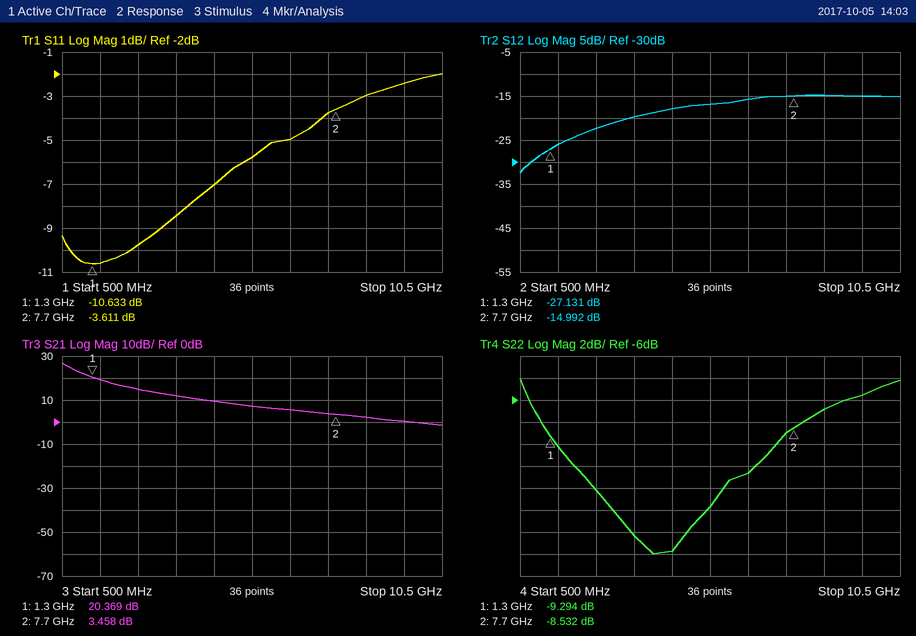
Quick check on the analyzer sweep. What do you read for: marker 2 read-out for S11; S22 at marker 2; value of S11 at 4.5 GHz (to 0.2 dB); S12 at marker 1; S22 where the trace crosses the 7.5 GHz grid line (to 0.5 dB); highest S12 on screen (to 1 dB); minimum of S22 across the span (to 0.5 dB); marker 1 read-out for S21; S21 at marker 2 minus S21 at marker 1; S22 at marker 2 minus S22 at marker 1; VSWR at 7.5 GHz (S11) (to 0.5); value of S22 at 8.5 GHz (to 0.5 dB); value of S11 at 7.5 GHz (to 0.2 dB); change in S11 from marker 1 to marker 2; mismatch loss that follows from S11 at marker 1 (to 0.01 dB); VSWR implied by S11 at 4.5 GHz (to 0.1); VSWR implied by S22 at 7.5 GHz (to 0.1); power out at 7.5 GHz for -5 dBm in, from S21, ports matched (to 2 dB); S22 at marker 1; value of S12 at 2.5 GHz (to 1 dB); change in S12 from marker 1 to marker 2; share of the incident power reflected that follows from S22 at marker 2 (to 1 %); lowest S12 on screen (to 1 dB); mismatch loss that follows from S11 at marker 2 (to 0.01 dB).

-3.611 dB
-8.532 dB
-7.0 dB
-27.131 dB
-9.0 dB
-15 dB
-20.0 dB
20.369 dB
-16.911 dB
0.762 dB
4.5
-7.0 dB
-3.8 dB
7.022 dB
0.39 dB
2.6
2.1
-2 dBm
-9.294 dB
-22 dB
12.139 dB
14 %
-32 dB
2.48 dB
